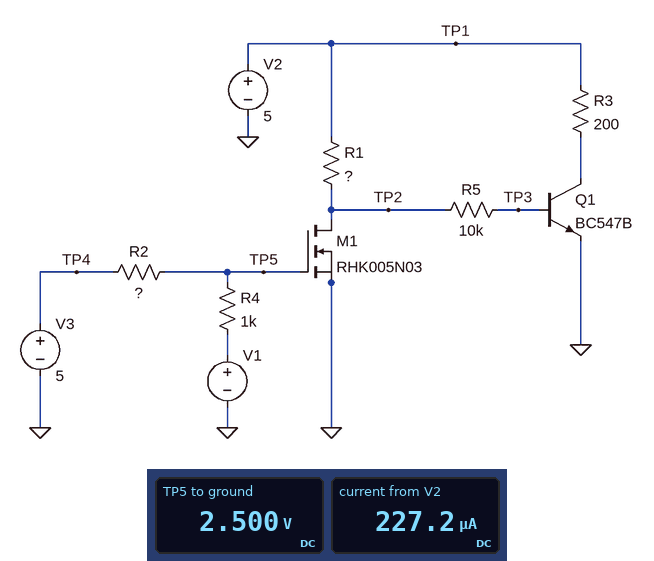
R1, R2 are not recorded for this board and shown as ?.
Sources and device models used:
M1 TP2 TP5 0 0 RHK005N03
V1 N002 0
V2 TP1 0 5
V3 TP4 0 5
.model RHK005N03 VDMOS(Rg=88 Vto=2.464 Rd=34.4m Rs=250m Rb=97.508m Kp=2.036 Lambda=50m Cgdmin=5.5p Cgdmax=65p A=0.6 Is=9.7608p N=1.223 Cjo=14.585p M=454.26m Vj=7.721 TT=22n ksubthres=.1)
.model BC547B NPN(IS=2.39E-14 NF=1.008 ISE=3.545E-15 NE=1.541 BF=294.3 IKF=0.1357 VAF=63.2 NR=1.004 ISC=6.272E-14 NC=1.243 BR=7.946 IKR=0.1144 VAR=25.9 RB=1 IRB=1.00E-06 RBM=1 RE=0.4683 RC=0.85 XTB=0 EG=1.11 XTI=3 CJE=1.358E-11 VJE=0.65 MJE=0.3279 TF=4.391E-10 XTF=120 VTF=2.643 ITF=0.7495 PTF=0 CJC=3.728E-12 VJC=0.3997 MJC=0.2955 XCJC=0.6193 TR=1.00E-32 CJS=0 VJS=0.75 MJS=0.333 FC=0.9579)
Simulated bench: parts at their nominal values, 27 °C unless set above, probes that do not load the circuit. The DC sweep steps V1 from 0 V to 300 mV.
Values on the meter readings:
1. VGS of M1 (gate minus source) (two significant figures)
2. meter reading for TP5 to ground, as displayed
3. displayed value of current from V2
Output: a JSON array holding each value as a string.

["2.5 V", "2.500 V", "227.2 µA"]
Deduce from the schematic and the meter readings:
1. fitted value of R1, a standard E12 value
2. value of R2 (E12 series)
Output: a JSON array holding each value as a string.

["22 kΩ", "1 kΩ"]
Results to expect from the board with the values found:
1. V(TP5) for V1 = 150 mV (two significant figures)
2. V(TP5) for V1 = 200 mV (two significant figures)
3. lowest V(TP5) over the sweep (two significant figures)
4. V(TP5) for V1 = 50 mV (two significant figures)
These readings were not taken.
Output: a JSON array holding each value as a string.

["2.6 V", "2.6 V", "2.5 V", "2.5 V"]
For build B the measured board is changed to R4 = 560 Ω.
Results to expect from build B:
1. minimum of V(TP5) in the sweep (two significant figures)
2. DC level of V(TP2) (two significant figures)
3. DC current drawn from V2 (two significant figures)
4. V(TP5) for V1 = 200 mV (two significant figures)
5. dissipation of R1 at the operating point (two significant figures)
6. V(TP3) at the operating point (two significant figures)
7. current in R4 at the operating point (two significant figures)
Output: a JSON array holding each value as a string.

["1.8 V", "2.1 V", "24 mA", "1.9 V", "390 µW", "740 mV", "3.2 mA"]
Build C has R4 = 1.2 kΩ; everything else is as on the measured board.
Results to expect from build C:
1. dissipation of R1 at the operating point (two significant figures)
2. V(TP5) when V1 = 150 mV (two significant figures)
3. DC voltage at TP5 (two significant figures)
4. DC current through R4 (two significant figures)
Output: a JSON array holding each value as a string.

["1.1 mW", "2.8 V", "2.7 V", "2.3 mA"]
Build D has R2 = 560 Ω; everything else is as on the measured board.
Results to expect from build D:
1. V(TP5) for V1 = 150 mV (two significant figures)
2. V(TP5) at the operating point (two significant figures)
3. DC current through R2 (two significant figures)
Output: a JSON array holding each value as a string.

["3.3 V", "3.2 V", "3.2 mA"]
